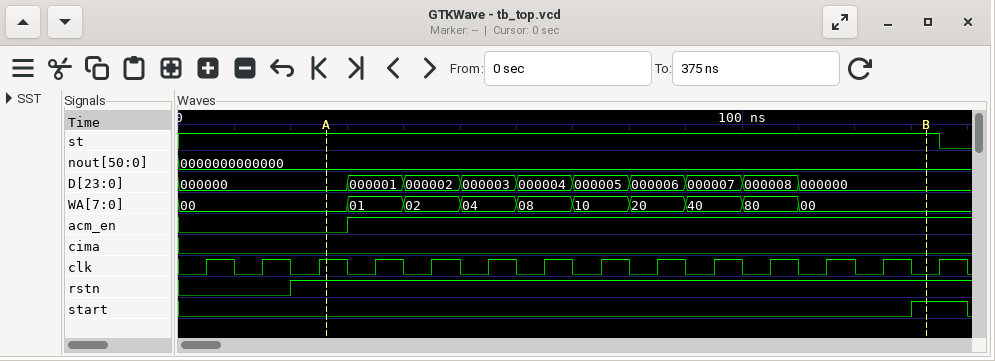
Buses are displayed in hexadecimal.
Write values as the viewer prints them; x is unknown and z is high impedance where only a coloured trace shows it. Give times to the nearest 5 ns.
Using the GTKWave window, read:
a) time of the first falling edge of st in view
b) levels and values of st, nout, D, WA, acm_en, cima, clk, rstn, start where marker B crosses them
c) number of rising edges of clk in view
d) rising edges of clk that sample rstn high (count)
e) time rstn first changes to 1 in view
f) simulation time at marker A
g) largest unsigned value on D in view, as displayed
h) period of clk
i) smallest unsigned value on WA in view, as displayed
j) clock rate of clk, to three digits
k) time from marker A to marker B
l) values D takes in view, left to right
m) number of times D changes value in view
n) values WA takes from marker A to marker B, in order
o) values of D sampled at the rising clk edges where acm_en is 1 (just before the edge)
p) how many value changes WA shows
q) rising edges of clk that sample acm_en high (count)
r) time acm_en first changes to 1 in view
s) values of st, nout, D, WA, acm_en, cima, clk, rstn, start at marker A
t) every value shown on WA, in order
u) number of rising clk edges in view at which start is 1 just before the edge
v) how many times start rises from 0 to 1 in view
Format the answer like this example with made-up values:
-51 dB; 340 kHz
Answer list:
135 ns; st=1, nout=0000000000000, D=000000, WA=00, acm_en=1, cima=0, clk=0, rstn=1, start=1; 14; 12; 20 ns; 25 ns; 000008; 10 ns; 00; 100 MHz; 105 ns; 000000, 000001, 000002, 000003, 000004, 000005, 000006, 000007, 000008, 000000; 9; 00, 01, 02, 04, 08, 10, 20, 40, 80, 00; 000001, 000002, 000003, 000004, 000005, 000006, 000007, 000008, 000000, 000000, 000000; 9; 11; 30 ns; st=1, nout=0000000000000, D=000000, WA=00, acm_en=0, cima=0, clk=1, rstn=1, start=0; 00, 01, 02, 04, 08, 10, 20, 40, 80, 00; 1; 1
